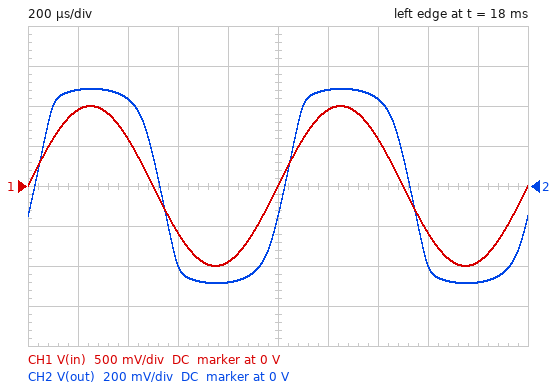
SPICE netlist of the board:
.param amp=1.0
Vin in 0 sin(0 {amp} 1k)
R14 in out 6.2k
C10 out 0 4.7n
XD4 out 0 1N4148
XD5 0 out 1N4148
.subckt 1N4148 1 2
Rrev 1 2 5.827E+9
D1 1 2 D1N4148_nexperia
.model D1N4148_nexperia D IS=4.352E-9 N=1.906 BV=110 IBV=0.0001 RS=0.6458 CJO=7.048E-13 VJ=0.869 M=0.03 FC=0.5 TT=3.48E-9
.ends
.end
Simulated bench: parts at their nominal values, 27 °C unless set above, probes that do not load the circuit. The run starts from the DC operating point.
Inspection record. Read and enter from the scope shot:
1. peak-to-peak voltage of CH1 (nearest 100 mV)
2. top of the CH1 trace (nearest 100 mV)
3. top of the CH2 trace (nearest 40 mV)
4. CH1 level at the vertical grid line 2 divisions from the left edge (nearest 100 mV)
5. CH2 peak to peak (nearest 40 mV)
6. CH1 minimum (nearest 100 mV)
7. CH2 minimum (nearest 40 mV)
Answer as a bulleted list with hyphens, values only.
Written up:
- 2.0 V
- 1.0 V
- 480 mV
- 600 mV
- 960 mV
- -1.0 V
- -480 mV
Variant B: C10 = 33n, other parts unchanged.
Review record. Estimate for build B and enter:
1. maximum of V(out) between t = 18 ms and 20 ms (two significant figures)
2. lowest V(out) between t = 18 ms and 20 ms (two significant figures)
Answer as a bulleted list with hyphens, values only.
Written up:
- 480 mV
- -480 mV
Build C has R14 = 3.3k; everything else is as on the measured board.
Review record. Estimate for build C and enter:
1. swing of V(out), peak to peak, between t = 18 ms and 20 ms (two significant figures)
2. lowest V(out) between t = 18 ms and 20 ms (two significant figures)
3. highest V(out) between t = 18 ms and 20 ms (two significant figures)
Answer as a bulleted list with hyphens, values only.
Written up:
- 1.0 V
- -510 mV
- 510 mV
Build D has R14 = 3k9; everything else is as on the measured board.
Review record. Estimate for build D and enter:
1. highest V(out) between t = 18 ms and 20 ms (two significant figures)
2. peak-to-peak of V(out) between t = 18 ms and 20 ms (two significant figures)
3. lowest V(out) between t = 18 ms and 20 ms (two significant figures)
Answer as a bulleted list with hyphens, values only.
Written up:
- 510 mV
- 1.0 V
- -510 mV
